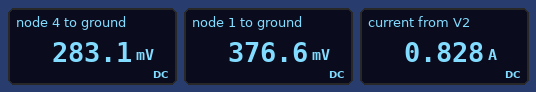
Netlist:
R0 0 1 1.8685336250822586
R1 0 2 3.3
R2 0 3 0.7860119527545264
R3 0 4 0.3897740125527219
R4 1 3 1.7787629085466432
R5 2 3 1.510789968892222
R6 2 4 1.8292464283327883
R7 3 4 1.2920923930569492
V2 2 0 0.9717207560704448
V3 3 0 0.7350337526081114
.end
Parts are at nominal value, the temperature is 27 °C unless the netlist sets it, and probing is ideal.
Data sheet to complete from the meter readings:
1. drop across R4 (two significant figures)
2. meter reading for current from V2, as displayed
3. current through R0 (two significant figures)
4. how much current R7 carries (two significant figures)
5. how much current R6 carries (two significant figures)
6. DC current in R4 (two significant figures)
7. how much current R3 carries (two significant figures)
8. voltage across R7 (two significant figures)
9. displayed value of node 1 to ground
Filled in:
360 mV
0.828 A
200 mA
350 mA
380 mA
200 mA
730 mA
450 mV
376.6 mV
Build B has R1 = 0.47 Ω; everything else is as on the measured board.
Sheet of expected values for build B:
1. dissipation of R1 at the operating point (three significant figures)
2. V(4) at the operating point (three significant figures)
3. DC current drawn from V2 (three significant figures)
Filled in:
2.01 W
283 mV
2.60 A
